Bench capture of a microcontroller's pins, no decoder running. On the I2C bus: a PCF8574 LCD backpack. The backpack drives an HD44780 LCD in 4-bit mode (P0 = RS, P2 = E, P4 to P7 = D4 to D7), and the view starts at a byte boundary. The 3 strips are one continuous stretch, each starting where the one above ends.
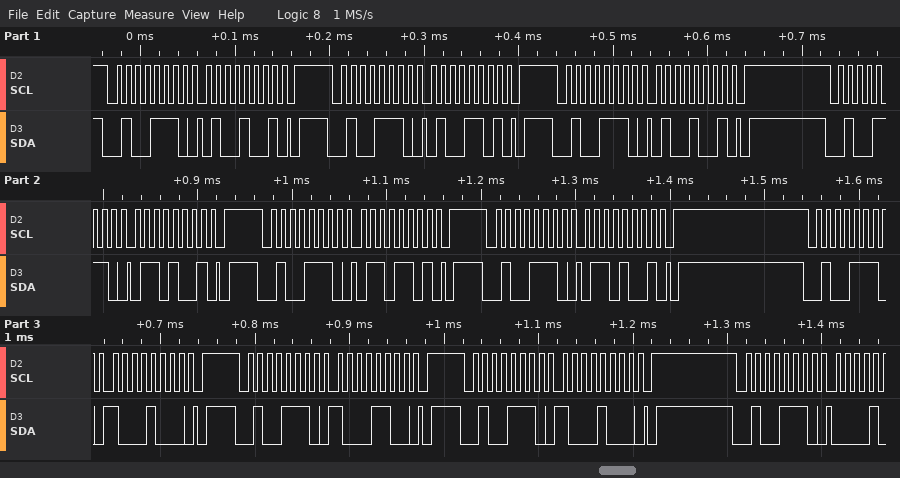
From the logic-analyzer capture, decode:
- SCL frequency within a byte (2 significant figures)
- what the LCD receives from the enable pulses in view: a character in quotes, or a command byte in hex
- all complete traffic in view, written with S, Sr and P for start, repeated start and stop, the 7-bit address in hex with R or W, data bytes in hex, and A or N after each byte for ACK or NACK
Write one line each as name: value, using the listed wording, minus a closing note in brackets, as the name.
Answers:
SCL frequency within a byte: 100 kHz
what the LCD receives from the enable pulses in view: a character in quotes, or a command byte in hex: 'F'
all complete traffic in view, written with S, Sr and P for start, repeated start and stop, the 7-bit address in hex with R or W, data bytes in hex, and A or N after each byte for ACK or NACK: S 27W A 49 A P S 27W A 4D A P S 27W A 49 A P S 27W A 69 A P S 27W A 6D A P S 27W A 69 A P S 27W A 88 A P S 27W A 8C A P S 27W A 88 A P S 27W A
